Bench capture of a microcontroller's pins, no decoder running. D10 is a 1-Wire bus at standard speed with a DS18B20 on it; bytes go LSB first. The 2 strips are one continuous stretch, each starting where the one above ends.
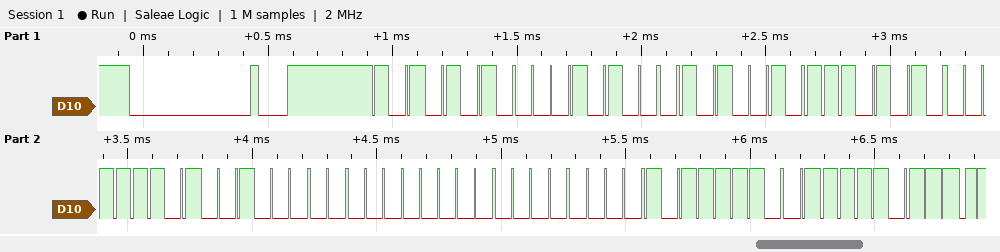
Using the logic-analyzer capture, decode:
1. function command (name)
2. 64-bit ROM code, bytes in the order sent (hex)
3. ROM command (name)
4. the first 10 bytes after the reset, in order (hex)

Read Scratchpad
28 4A 57 BC 04 00 00 7D
Match ROM
55 28 4A 57 BC 04 00 00 7D BE
